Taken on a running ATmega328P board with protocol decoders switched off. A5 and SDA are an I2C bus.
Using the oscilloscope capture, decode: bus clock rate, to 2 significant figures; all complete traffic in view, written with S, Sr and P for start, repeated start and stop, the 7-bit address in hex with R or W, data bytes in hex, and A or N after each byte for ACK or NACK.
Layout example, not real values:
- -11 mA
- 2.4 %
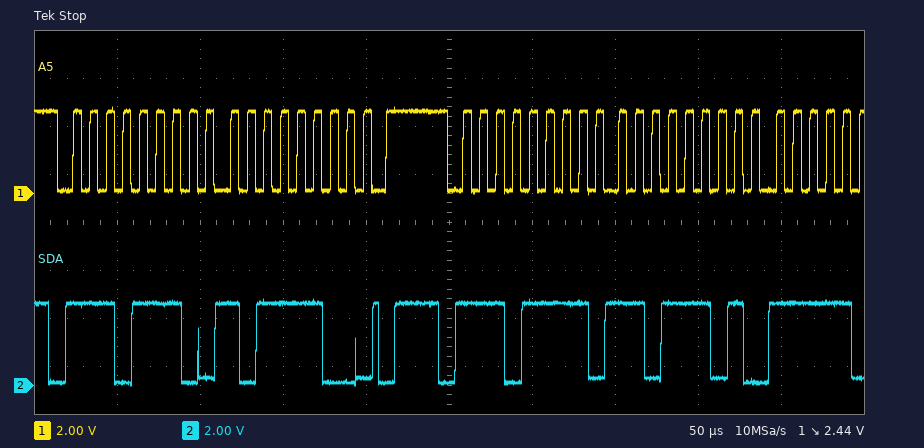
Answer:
- 100 kHz
- S 77W A BC A P S 77R A DD A
